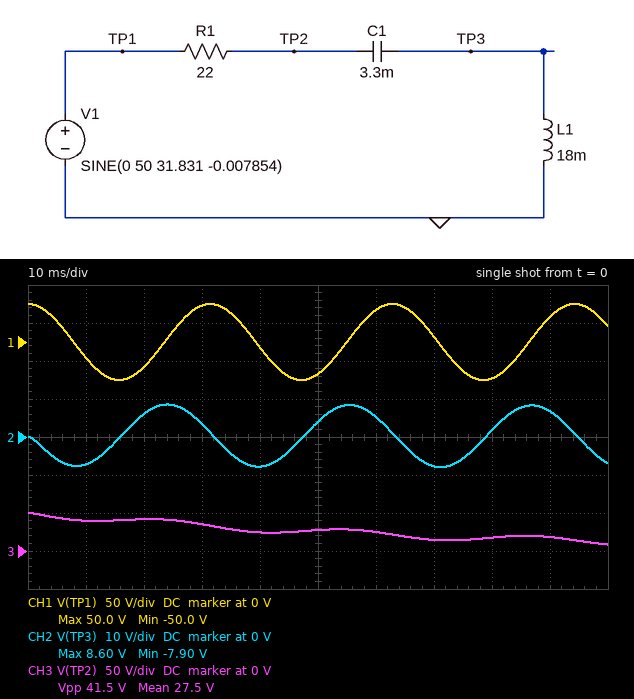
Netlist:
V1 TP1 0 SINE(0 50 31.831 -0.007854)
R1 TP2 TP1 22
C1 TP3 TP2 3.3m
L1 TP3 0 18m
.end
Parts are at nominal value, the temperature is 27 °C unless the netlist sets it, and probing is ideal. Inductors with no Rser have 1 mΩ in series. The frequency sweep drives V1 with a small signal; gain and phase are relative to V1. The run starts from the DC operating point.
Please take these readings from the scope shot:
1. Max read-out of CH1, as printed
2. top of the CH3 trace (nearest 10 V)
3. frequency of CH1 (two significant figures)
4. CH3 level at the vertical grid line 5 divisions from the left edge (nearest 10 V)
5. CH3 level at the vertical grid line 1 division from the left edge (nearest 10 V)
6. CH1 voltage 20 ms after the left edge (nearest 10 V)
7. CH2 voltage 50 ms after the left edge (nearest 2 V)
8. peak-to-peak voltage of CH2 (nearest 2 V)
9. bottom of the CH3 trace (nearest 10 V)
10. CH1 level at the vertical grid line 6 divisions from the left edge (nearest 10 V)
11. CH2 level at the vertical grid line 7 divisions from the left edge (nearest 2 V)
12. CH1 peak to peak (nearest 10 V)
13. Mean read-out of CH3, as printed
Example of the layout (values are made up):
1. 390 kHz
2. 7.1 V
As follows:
1. 50.0 V
2. 50 V
3. 32 Hz
4. 30 V
5. 40 V
6. -30 V
7. 4 V
8. 16 V
9. 10 V
10. 40 V
11. -8 V
12. 100 V
13. 27.5 V
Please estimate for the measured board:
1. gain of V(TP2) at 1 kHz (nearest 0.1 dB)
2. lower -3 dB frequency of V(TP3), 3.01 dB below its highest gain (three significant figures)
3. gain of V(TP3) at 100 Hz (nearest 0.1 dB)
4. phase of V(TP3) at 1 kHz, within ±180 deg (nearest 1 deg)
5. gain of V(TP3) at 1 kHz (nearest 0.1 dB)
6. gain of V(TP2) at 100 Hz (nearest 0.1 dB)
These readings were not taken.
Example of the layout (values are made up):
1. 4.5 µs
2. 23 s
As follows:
1. -0.2 dB
2. 192 Hz
3. -6.7 dB
4. 11 deg
5. -0.2 dB
6. -7.1 dB
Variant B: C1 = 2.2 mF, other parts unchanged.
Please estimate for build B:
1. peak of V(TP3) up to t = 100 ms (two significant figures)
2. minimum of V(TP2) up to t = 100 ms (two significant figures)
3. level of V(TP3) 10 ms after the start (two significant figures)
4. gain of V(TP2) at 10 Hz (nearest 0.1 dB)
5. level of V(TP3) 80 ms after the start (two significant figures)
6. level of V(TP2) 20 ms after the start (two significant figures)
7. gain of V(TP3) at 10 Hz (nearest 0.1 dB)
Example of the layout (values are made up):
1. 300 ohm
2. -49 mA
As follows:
1. 8.7 V
2. 3.6 V
3. -6.9 V
4. -11.5 dB
5. 2.0 V
6. 36 V
7. -26.1 dB
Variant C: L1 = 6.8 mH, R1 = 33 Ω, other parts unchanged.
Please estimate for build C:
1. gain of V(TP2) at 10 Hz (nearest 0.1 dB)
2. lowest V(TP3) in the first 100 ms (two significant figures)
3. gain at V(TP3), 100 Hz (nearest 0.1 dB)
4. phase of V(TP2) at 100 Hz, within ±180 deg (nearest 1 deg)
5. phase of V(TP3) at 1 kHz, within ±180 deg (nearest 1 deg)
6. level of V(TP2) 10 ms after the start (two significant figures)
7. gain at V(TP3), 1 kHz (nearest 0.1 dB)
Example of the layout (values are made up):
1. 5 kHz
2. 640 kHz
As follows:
1. -17.6 dB
2. -2.0 V
3. -17.8 dB
4. 83 deg
5. 38 deg
6. 46 V
7. -2.0 dB
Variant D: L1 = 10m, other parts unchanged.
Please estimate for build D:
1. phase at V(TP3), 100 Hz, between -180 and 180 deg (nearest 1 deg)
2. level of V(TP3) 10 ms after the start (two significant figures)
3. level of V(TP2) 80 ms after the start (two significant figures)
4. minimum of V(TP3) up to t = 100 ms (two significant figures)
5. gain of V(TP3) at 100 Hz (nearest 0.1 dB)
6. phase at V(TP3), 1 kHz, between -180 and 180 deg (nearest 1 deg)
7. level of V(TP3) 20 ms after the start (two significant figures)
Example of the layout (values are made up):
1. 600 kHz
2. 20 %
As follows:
1. 75 deg
2. -3.9 V
3. 17 V
4. -4.4 V
5. -11.2 dB
6. 19 deg
7. 3.6 V
